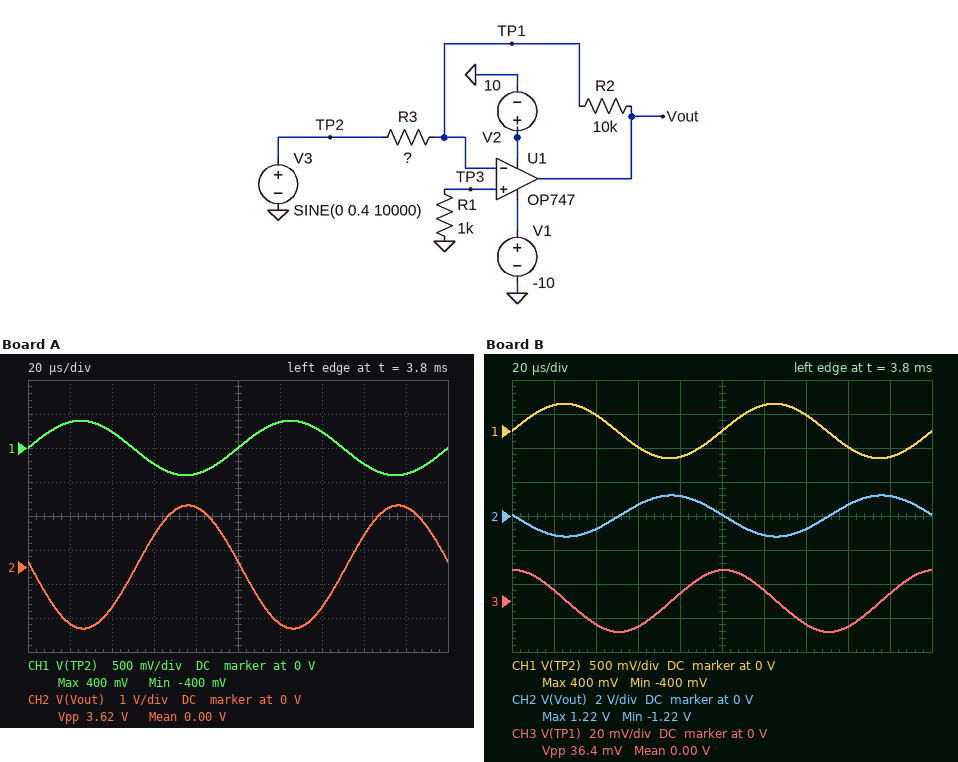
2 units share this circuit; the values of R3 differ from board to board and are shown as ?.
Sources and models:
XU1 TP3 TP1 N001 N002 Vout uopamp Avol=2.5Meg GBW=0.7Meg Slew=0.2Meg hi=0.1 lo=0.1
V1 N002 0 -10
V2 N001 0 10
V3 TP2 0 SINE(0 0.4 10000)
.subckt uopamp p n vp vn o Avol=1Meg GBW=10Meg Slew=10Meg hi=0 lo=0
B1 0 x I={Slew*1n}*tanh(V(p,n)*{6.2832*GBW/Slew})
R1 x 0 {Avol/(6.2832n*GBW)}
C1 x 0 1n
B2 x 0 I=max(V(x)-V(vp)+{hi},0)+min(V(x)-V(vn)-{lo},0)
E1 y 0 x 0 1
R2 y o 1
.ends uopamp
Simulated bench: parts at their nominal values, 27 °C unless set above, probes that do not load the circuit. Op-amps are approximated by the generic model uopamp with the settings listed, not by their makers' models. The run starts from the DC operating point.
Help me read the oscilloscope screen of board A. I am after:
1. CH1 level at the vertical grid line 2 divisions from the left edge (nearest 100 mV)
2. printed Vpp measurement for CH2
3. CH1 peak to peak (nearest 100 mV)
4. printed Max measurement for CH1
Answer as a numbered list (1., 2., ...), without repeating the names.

1. 200 mV
2. 3.62 V
3. 800 mV
4. 400 mV
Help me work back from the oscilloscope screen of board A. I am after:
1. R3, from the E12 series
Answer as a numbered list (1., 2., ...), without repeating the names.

1. 2.2 kΩ
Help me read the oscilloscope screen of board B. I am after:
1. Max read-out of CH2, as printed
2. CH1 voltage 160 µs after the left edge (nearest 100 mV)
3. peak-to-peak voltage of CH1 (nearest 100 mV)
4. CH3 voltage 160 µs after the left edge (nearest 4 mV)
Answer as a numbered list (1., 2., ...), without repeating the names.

1. 1.22 V
2. -200 mV
3. 800 mV
4. -16 mV
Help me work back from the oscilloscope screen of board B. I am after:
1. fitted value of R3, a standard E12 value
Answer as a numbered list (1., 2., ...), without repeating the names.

1. 3.3 kΩ
